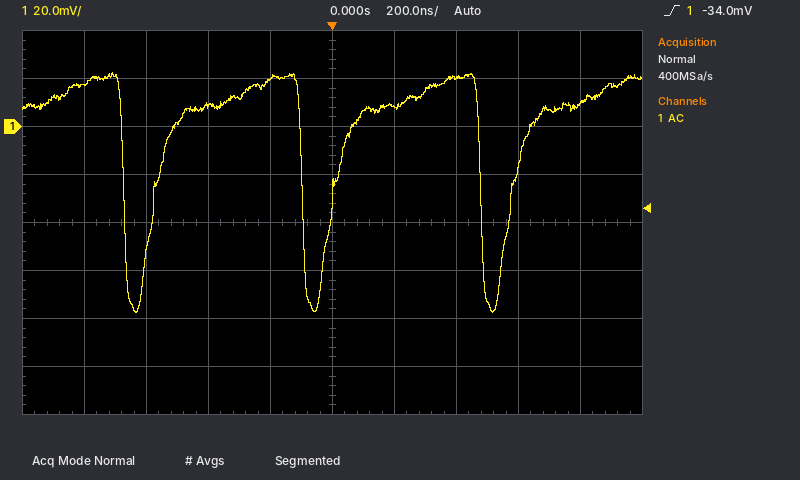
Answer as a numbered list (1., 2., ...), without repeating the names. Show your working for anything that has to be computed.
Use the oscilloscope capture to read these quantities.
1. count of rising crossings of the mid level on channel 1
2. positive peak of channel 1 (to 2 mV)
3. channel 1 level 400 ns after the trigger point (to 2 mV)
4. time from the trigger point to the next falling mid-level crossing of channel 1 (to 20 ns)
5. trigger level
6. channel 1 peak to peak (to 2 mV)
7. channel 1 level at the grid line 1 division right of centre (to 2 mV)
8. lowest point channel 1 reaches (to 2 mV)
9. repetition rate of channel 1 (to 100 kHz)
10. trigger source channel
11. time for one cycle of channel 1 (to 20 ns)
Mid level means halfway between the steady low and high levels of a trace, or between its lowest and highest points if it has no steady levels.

1. 3
2. 22 mV
3. 20 mV
4. 480 ns
5. -34.0 mV
6. 22 mV − (-78 mV) = 100 mV
7. 8 mV
8. -78 mV
9. 1 / 580 ns ≈ 1.7 MHz
10. channel 1
11. 580 ns
